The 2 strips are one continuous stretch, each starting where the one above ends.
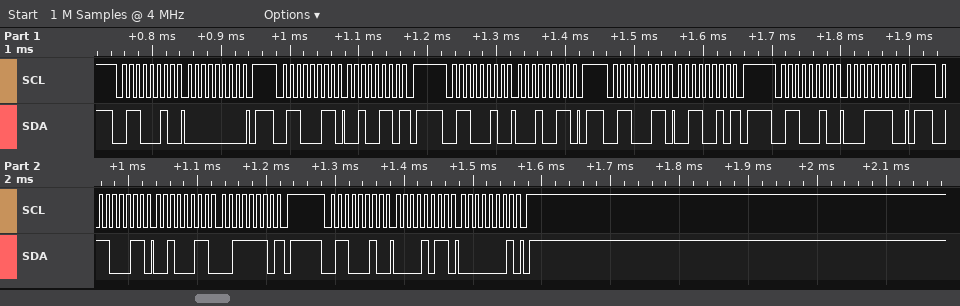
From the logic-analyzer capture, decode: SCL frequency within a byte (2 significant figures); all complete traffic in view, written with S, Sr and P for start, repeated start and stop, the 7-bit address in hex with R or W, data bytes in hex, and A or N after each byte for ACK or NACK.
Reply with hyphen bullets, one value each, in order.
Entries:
- 100 kHz
- S 31W A 00 A P S 31R A 26 N P S 31W A 13 A P S 31R A 32 N P S 31W A 1E A P S 31R A 23 A 3E N P S 31W A 0B A 01 A P
